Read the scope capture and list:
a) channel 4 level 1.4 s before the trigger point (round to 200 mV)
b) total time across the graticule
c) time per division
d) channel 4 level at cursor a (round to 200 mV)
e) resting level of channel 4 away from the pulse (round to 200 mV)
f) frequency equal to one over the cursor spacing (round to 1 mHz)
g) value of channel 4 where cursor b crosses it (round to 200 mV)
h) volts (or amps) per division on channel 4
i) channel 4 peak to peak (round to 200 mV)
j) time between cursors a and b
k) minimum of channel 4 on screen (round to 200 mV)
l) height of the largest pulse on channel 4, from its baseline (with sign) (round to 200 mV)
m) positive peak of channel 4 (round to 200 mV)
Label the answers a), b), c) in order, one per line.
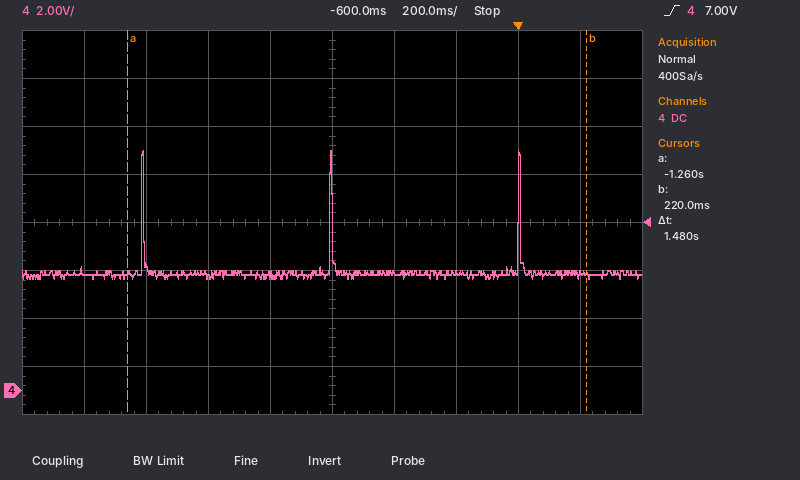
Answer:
a) 5.0 V
b) 2 s
c) 200 ms
d) 4.8 V
e) 4.8 V
f) 676 mHz
g) 4.8 V
h) 2 V
i) 5.4 V
j) 1.48 s
k) 4.6 V
l) +5.2 V
m) 10.0 V
